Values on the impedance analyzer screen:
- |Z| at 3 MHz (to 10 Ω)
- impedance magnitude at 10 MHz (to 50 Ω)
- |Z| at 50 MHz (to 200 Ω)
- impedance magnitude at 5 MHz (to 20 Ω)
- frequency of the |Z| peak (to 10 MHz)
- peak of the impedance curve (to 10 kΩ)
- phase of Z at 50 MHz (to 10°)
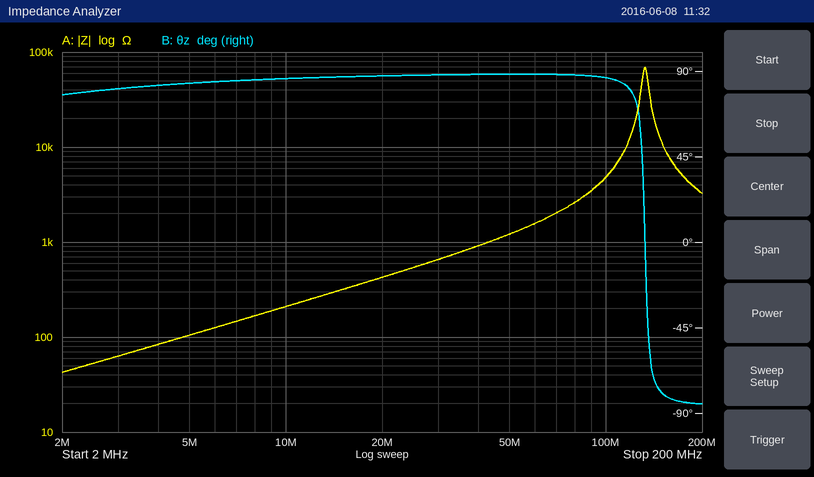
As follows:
60 Ω
200 Ω
1.2 kΩ
100 Ω
130 MHz
70 kΩ
90°
